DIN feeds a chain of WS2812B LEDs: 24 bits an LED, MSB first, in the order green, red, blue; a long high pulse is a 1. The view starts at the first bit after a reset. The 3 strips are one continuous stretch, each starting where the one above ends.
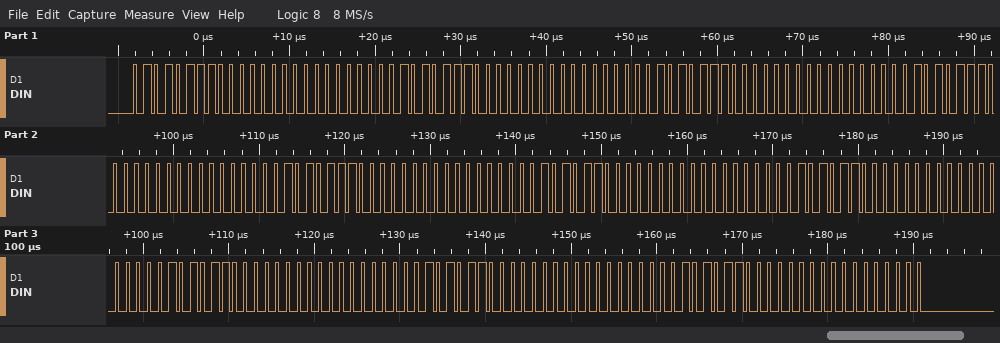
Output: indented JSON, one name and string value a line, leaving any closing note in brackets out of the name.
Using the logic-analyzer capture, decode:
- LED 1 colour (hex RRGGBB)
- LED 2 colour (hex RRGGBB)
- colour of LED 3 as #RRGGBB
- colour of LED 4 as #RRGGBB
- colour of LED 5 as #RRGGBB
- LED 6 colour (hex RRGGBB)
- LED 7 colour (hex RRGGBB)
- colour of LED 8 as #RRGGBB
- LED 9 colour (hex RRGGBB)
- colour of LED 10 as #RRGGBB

{
  "LED 1 colour": "#005700",
  "LED 2 colour": "#005700",
  "colour of LED 3 as #RRGGBB": "#005700",
  "colour of LED 4 as #RRGGBB": "#005700",
  "colour of LED 5 as #RRGGBB": "#005700",
  "LED 6 colour": "#005600",
  "LED 7 colour": "#005600",
  "colour of LED 8 as #RRGGBB": "#005600",
  "LED 9 colour": "#005600",
  "colour of LED 10 as #RRGGBB": "#005600"
}
